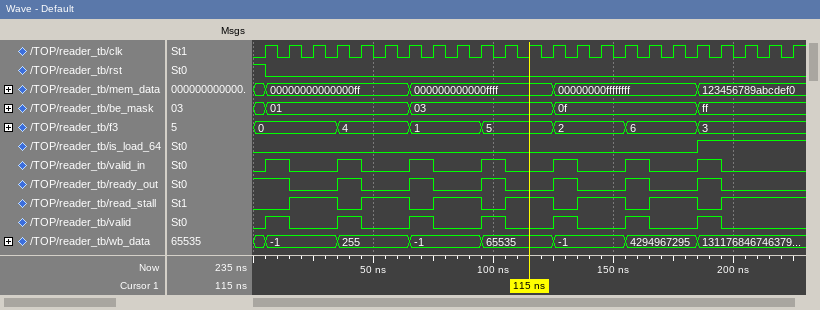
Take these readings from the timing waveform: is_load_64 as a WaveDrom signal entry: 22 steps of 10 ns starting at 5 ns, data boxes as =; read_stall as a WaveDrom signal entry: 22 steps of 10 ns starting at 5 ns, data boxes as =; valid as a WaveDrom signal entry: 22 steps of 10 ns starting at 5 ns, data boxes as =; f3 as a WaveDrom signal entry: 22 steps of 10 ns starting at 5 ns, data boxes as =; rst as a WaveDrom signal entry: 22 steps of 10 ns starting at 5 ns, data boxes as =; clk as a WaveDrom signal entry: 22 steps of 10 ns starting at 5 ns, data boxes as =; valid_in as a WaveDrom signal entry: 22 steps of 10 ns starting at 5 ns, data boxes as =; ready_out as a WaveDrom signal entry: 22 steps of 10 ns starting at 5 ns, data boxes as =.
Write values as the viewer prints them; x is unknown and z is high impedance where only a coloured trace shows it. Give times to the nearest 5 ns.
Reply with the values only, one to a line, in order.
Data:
{name: 'is_load_64', wave: '0.................1...'}
{name: 'read_stall', wave: '01.01.01.01.01.01.01..'}
{name: 'valid', wave: '10.10.10.10.10.10.10..'}
{name: 'f3', wave: '=..=..=..=..=..=..=...', data: '0 4 1 5 2 6 3'}
{name: 'rst', wave: '0.....................'}
{name: 'clk', wave: 'p.....................'}
{name: 'valid_in', wave: '10.10.10.10.10.10.10..'}
{name: 'ready_out', wave: '10.10.10.10.10.10.10..'}
